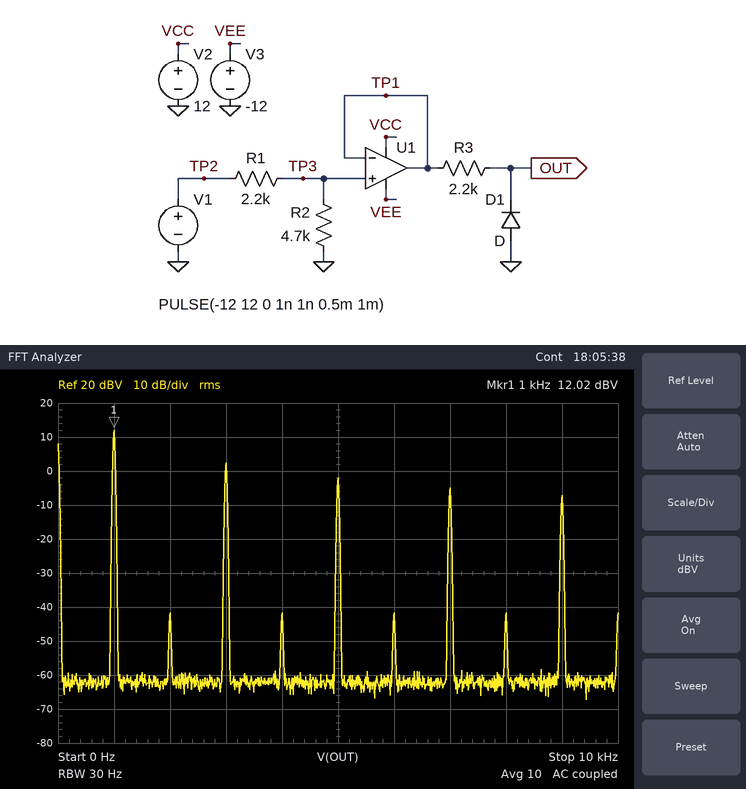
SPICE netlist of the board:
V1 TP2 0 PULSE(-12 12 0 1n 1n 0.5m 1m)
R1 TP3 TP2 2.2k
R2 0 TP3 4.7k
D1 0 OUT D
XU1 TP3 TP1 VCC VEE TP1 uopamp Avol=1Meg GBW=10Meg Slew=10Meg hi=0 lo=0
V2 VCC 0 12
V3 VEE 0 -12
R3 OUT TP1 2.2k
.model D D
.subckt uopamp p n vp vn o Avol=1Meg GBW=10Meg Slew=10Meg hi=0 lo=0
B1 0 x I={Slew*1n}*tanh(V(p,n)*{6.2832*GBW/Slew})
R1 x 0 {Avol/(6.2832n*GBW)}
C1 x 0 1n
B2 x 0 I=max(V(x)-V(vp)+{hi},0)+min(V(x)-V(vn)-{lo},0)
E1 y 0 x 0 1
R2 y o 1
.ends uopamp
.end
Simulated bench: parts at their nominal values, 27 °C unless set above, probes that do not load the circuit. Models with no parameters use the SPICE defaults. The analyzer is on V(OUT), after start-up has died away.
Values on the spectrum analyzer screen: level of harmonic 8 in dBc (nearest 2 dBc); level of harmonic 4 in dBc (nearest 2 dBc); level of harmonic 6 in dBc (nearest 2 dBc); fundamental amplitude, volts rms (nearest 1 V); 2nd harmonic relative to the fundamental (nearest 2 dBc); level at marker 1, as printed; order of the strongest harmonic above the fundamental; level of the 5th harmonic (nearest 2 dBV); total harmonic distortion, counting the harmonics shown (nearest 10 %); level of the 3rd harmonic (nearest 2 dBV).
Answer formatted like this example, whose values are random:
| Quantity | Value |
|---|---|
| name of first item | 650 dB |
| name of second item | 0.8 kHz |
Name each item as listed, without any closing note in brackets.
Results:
| Quantity | Value |
|---|---|
| level of harmonic 8 in dBc | -54 dBc |
| level of harmonic 4 in dBc | -54 dBc |
| level of harmonic 6 in dBc | -54 dBc |
| fundamental amplitude, volts rms | 4 V |
| 2nd harmonic relative to the fundamental | -54 dBc |
| level at marker 1, as printed | 12.02 dBV |
| order of the strongest harmonic above the fundamental | 3 |
| level of the 5th harmonic | -2 dBV |
| total harmonic distortion, counting the harmonics shown | 40 % |
| level of the 3rd harmonic | 2 dBV |
